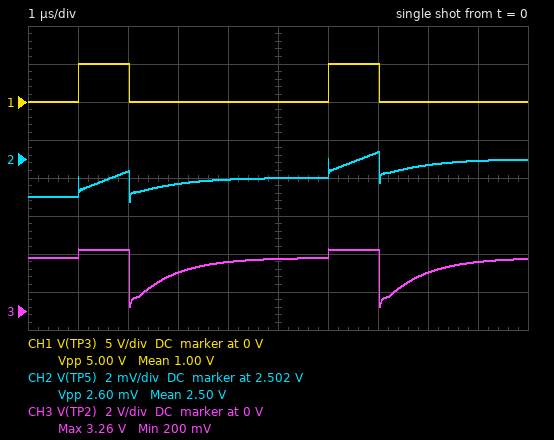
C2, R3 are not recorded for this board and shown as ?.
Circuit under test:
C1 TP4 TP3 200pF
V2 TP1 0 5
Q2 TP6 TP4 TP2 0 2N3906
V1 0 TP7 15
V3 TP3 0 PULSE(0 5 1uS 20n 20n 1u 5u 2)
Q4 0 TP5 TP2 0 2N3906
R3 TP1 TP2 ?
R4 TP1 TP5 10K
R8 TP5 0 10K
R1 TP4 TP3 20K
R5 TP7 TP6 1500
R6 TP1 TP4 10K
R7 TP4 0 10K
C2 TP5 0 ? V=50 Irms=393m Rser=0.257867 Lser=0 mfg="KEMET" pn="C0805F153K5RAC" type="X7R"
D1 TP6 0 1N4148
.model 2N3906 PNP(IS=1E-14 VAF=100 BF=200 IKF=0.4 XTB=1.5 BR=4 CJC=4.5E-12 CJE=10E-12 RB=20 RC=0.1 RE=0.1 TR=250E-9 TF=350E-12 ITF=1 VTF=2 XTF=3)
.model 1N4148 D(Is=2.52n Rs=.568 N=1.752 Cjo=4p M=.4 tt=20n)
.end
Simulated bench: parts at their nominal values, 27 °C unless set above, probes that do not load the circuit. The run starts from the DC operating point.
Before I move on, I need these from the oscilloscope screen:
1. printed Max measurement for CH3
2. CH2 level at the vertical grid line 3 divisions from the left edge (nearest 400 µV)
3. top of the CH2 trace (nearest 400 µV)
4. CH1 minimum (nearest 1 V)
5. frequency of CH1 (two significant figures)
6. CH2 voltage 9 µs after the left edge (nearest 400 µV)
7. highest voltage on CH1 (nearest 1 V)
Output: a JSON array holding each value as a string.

["3.26 V", "2.5008 V", "2.5024 V", "0 V", "200 kHz", "2.5020 V", "5 V"]
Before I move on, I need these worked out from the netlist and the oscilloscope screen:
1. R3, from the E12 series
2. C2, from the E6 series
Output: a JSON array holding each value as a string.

["390 Ω", "22 nF"]
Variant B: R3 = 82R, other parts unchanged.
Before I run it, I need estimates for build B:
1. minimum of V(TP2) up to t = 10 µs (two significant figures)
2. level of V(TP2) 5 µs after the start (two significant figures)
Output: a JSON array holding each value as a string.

["870 mV", "3.2 V"]
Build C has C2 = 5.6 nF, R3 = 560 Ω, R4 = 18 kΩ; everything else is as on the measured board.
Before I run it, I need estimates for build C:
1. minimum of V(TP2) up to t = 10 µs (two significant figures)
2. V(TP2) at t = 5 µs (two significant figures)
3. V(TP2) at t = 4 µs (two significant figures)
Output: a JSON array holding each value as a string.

["130 mV", "2.6 V", "2.5 V"]
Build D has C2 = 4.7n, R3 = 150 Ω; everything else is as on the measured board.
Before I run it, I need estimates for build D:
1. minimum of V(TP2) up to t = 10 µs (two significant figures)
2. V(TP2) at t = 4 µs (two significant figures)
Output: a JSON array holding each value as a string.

["770 mV", "2.8 V"]
